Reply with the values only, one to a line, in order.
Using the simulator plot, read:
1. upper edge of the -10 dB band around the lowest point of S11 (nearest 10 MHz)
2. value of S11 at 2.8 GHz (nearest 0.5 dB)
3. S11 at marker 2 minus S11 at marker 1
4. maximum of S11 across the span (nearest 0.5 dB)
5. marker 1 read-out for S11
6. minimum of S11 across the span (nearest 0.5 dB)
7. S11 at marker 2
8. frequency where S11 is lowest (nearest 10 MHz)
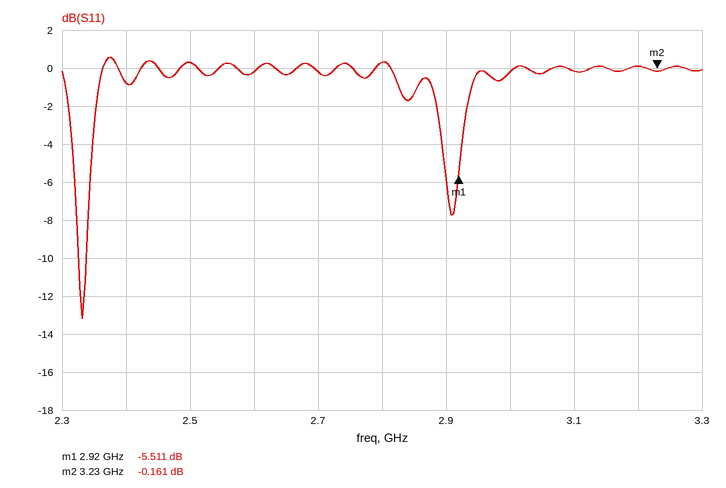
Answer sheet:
2.34 GHz
0.5 dB
5.350 dB
0.5 dB
-5.511 dB
-13.0 dB
-0.161 dB
2.33 GHz
